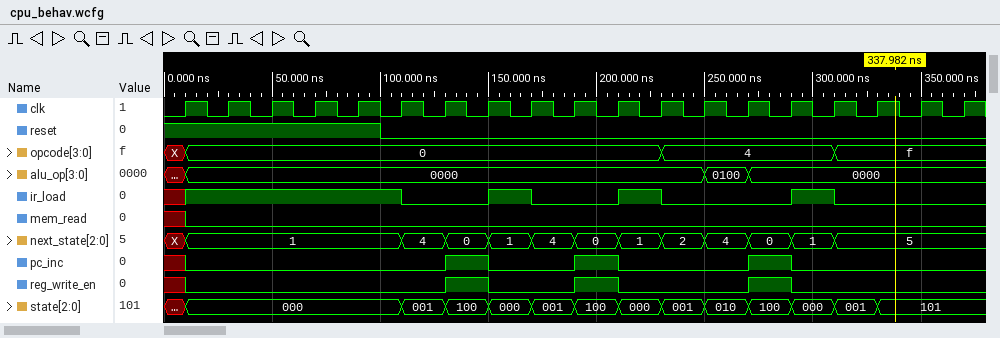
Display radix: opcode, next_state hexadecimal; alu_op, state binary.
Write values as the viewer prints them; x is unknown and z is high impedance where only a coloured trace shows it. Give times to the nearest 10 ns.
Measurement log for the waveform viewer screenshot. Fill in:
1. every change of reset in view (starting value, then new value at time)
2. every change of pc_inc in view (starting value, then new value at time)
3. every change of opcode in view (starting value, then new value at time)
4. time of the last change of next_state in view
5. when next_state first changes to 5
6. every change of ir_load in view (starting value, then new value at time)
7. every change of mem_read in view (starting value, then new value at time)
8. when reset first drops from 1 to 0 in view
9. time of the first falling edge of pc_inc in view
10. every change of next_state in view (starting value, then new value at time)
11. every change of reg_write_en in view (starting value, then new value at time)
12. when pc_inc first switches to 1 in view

1, 0 at 100 ns
x, 0 at 10 ns, 1 at 130 ns, 0 at 150 ns, 1 at 190 ns, 0 at 210 ns, 1 at 270 ns, 0 at 290 ns
X, 0 at 10 ns, 4 at 230 ns, f at 310 ns
310 ns
310 ns
x, 1 at 10 ns, 0 at 110 ns, 1 at 150 ns, 0 at 170 ns, 1 at 210 ns, 0 at 230 ns, 1 at 290 ns, 0 at 310 ns
x, 0 at 10 ns
100 ns
150 ns
X, 1 at 10 ns, 4 at 110 ns, 0 at 130 ns, 1 at 150 ns, 4 at 170 ns, 0 at 190 ns, 1 at 210 ns, 2 at 230 ns, 4 at 250 ns, 0 at 270 ns, 1 at 290 ns, 5 at 310 ns
x, 0 at 10 ns, 1 at 130 ns, 0 at 150 ns, 1 at 190 ns, 0 at 210 ns, 1 at 270 ns, 0 at 290 ns
130 ns
